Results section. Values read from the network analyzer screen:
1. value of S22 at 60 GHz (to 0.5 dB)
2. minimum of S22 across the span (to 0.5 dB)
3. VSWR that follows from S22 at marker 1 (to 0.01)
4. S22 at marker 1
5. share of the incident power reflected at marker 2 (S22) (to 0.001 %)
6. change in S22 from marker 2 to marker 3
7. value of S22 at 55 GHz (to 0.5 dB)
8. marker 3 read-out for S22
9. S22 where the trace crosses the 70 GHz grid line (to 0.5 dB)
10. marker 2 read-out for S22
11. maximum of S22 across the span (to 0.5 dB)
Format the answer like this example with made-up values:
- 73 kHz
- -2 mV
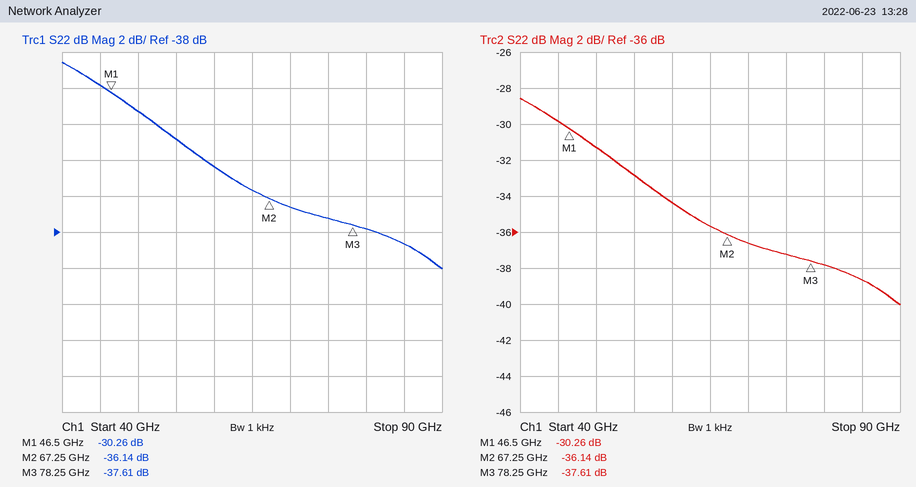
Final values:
- -34.5 dB
- -40.0 dB
- 1.06
- -30.26 dB
- 0.024 %
- -1.47 dB
- -33.0 dB
- -37.61 dB
- -36.5 dB
- -36.14 dB
- -28.5 dB
